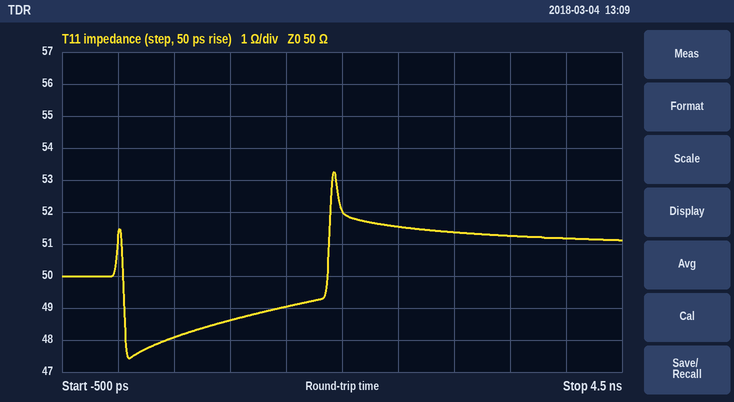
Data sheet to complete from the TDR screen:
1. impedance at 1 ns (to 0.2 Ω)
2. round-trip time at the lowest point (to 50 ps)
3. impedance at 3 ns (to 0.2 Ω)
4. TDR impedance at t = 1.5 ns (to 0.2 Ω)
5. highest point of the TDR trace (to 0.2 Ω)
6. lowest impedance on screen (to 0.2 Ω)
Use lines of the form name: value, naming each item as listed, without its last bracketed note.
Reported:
impedance at 1 ns: 48.6 Ω
round-trip time at the lowest point: 100 ps
impedance at 3 ns: 51.4 Ω
TDR impedance at t = 1.5 ns: 49.0 Ω
highest point of the TDR trace: 53.2 Ω
lowest impedance on screen: 47.4 Ω
